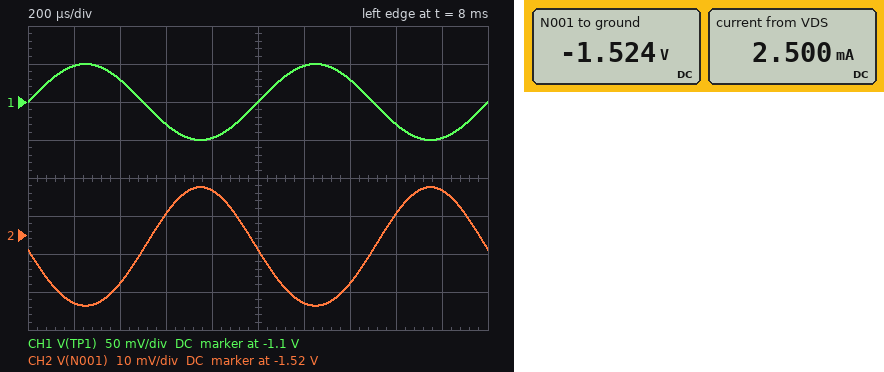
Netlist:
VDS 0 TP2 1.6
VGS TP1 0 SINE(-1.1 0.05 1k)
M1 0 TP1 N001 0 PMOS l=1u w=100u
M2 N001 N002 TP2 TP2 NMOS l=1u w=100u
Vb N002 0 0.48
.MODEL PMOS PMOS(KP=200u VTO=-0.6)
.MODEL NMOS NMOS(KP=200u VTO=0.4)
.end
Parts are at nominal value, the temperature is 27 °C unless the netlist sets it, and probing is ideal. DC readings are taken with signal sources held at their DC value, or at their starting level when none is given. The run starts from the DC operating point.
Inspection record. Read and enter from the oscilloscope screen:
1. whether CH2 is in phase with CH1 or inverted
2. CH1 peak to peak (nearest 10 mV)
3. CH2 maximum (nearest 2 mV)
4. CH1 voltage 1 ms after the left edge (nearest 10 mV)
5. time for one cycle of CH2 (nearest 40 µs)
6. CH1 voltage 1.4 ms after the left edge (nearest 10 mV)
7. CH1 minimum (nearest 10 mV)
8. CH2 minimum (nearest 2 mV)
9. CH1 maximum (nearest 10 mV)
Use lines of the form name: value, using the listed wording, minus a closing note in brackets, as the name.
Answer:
whether CH2 is in phase with CH1 or inverted: inverted
CH1 peak to peak: 100 mV
CH2 maximum: -1.508 V
CH1 voltage 1 ms after the left edge: -1.10 V
time for one cycle of CH2: 1.00 ms
CH1 voltage 1.4 ms after the left edge: -1.07 V
CH1 minimum: -1.15 V
CH2 minimum: -1.538 V
CH1 maximum: -1.05 V
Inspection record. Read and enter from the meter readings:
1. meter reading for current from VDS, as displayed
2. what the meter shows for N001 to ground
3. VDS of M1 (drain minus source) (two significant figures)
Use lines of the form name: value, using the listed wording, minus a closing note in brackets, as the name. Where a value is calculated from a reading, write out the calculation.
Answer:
meter reading for current from VDS, as displayed: 2.500 mA
what the meter shows for N001 to ground: -1.524 V
VDS of M1 (drain minus source): 0 V - (-1.524 V) = 1.5 V
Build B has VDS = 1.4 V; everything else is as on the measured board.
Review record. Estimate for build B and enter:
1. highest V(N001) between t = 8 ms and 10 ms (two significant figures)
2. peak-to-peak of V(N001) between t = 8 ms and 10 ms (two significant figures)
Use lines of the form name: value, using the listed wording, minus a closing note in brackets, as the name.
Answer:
highest V(N001) between t = 8 ms and 10 ms: -1.3 V
peak-to-peak of V(N001) between t = 8 ms and 10 ms: 36 mV
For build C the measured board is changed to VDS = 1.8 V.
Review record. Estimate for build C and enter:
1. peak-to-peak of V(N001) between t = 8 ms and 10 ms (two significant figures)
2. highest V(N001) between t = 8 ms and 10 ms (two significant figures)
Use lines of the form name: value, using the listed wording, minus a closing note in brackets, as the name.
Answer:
peak-to-peak of V(N001) between t = 8 ms and 10 ms: 28 mV
highest V(N001) between t = 8 ms and 10 ms: -1.7 V
